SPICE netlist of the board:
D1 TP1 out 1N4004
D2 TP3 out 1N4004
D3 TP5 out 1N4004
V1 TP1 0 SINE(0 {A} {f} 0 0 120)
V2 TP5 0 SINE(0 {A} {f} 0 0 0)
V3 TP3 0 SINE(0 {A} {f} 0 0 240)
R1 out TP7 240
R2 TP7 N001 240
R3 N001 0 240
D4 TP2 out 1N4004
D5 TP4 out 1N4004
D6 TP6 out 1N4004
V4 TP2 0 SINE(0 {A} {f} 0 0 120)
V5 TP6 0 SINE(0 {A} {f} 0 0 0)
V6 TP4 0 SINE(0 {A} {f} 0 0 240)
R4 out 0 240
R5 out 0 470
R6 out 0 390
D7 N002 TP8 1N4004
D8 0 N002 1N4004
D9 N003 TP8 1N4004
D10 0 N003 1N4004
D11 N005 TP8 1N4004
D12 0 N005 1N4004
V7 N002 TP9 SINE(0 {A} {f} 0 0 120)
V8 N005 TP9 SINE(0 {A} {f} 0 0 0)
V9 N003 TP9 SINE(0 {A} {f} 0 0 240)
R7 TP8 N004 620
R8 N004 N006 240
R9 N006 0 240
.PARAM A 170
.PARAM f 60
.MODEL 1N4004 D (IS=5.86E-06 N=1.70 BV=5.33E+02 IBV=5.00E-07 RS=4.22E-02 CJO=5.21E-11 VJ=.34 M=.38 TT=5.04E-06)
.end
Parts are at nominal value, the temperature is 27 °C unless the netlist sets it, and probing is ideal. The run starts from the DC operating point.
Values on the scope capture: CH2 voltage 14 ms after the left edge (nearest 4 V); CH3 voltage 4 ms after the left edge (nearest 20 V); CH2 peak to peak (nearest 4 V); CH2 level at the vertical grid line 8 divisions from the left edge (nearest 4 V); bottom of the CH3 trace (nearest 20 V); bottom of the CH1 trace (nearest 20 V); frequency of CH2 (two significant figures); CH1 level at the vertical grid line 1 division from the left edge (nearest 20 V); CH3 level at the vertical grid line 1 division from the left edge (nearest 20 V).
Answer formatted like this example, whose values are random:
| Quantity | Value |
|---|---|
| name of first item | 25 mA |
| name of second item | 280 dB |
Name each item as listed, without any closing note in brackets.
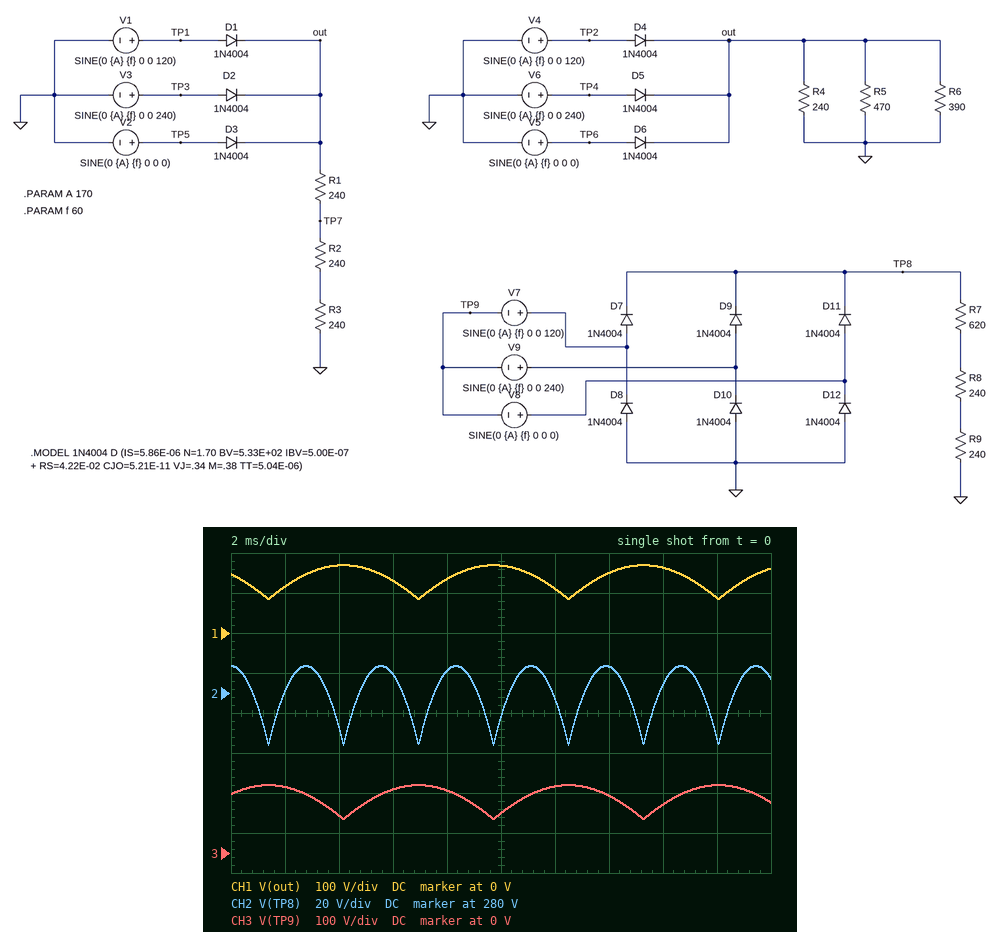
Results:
| Quantity | Value |
|---|---|
| CH2 voltage 14 ms after the left edge | 292 V |
| CH3 voltage 4 ms after the left edge | 100 V |
| CH2 peak to peak | 40 V |
| CH2 level at the vertical grid line 8 divisions from the left edge | 284 V |
| bottom of the CH3 trace | 80 V |
| bottom of the CH1 trace | 80 V |
| frequency of CH2 | 360 Hz |
| CH1 level at the vertical grid line 1 division from the left edge | 120 V |
| CH3 level at the vertical grid line 1 division from the left edge | 160 V |
